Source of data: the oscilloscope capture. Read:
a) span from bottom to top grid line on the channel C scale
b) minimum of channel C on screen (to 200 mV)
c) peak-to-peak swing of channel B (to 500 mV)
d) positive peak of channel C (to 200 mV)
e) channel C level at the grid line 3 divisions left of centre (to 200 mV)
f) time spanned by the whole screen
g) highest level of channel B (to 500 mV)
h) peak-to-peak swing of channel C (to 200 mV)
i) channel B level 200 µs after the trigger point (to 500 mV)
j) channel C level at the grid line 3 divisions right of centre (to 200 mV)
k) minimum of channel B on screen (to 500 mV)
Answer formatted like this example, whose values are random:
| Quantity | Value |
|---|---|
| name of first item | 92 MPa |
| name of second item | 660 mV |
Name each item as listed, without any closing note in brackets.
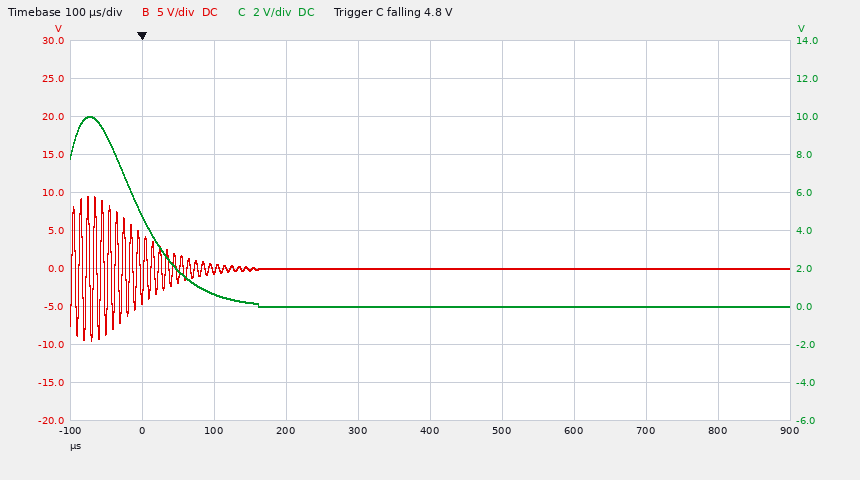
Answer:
| Quantity | Value |
|---|---|
| span from bottom to top grid line on the channel C scale | 20 V |
| minimum of channel C on screen | 0.0 V |
| peak-to-peak swing of channel B | 19.0 V |
| positive peak of channel C | 10.0 V |
| channel C level at the grid line 3 divisions left of centre | 600 mV |
| time spanned by the whole screen | 1 ms |
| highest level of channel B | 9.5 V |
| peak-to-peak swing of channel C | 10.0 V |
| channel B level 200 µs after the trigger point | 0.0 V |
| channel C level at the grid line 3 divisions right of centre | 0.0 V |
| minimum of channel B on screen | -9.5 V |
